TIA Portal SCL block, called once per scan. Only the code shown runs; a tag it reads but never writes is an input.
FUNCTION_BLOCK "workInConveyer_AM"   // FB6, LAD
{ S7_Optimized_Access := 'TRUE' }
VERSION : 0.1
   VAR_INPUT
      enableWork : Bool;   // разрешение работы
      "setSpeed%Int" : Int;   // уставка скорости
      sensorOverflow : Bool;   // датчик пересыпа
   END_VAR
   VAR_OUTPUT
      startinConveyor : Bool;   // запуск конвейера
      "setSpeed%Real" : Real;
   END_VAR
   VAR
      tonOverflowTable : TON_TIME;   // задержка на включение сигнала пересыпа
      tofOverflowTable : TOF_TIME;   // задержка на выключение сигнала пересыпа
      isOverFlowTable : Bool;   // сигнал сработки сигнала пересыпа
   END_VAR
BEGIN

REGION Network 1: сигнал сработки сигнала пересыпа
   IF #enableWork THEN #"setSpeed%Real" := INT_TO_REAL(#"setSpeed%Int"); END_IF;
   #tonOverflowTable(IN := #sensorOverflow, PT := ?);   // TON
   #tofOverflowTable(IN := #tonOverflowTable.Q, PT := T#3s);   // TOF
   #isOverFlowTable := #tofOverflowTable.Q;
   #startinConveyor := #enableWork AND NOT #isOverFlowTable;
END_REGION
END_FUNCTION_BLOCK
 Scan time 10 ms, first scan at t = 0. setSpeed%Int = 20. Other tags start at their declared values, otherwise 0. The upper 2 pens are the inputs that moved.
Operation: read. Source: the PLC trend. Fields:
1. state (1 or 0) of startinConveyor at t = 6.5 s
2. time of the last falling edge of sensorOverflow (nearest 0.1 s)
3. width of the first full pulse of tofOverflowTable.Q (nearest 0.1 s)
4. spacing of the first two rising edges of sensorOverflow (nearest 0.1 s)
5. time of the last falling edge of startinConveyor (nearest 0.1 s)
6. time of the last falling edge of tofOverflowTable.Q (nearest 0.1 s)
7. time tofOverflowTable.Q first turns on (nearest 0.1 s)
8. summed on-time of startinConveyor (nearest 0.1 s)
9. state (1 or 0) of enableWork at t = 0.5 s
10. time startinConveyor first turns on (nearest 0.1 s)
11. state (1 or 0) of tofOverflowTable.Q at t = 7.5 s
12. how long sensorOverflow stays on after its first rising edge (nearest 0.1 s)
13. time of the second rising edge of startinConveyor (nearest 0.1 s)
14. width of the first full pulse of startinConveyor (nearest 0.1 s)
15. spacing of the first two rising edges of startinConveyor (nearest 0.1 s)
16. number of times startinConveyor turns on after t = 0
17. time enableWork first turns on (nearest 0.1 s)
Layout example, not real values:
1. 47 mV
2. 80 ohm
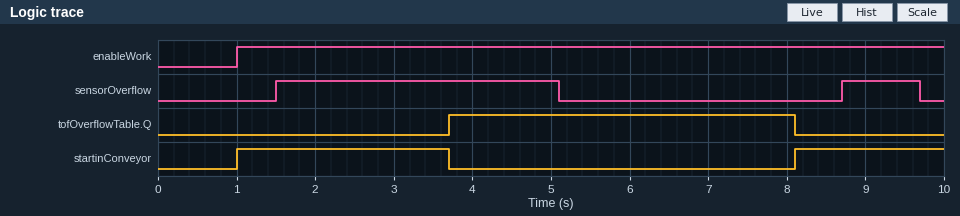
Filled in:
1. 0
2. 9.7 s
3. 4.4 s
4. 7.2 s
5. 3.7 s
6. 8.1 s
7. 3.7 s
8. 4.6 s
9. 0
10. 1.0 s
11. 1
12. 3.6 s
13. 8.1 s
14. 2.7 s
15. 7.1 s
16. 2
17. 1.0 s
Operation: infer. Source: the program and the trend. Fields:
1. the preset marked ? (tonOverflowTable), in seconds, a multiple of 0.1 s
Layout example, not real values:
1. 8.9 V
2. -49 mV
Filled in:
1. 2.2 s
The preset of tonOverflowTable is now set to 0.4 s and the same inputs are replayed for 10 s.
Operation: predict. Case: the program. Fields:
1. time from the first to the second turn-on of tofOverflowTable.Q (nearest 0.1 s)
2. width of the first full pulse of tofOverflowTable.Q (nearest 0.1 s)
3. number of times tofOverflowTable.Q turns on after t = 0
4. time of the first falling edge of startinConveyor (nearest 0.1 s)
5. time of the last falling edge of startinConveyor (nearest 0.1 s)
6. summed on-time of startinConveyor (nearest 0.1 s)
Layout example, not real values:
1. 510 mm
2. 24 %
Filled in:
1. 7.2 s
2. 6.2 s
3. 2
4. 1.9 s
5. 9.1 s
6. 1.9 s
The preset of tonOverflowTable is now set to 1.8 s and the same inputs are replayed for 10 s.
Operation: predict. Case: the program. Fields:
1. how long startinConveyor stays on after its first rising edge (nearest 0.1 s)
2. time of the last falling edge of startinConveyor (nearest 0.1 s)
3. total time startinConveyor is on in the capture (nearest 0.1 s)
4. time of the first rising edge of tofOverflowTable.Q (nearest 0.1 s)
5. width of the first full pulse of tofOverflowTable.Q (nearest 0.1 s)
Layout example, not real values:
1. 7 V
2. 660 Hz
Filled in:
1. 2.3 s
2. 3.3 s
3. 4.2 s
4. 3.3 s
5. 4.8 s
